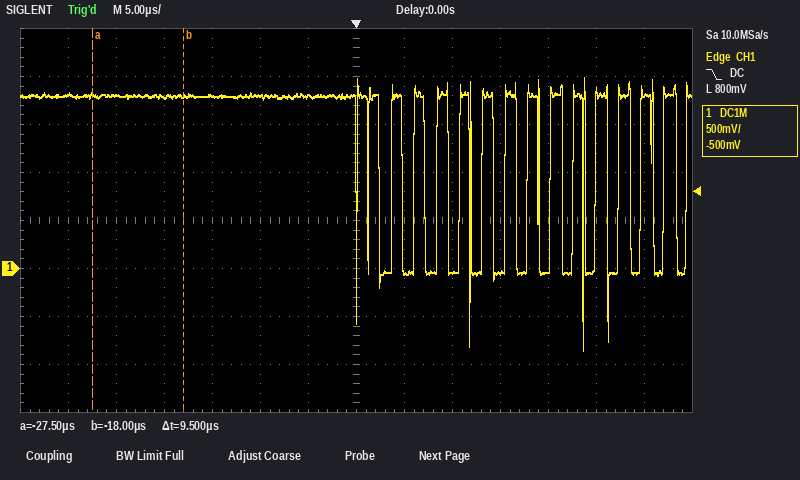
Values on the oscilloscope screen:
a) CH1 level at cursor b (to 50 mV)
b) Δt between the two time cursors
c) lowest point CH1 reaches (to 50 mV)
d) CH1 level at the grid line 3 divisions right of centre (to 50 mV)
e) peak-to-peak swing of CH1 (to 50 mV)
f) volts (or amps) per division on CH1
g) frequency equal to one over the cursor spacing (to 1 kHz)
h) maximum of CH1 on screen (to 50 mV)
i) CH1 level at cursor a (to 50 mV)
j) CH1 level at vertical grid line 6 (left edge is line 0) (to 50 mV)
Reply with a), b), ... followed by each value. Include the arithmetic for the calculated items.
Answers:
a) 1.80 V
b) 9.5 µs
c) -850 mV
d) -50 mV
e) 2.00 V − (-850 mV) = 2.85 V
f) 500 mV
g) 1 / 9.5 µs ≈ 105 kHz
h) 2.00 V
i) 1.80 V
j) 1.80 V
